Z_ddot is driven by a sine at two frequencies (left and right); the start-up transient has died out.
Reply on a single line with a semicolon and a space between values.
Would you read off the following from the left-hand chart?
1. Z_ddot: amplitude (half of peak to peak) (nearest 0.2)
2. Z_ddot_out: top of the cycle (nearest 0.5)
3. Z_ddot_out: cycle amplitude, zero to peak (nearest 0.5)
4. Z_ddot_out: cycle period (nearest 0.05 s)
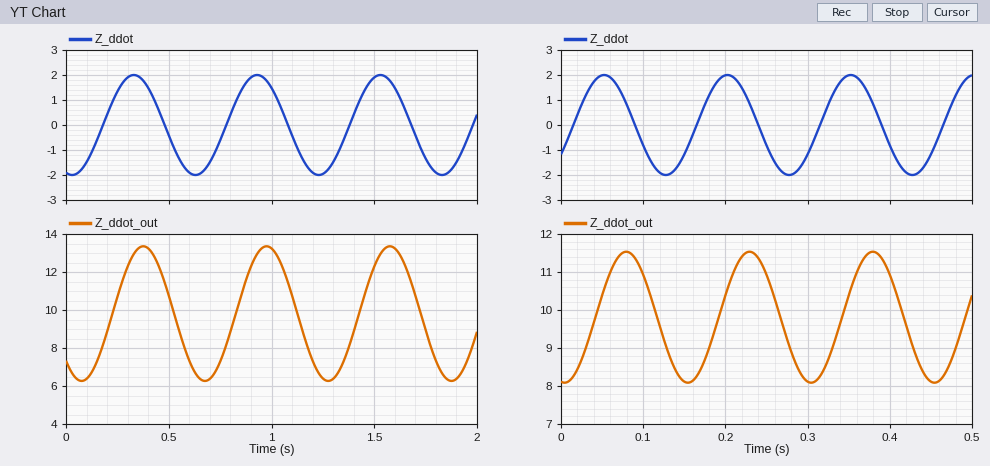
2.0; 13.5; 3.5; 0.60 s
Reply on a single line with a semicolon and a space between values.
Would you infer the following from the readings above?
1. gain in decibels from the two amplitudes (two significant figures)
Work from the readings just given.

4.9 dB
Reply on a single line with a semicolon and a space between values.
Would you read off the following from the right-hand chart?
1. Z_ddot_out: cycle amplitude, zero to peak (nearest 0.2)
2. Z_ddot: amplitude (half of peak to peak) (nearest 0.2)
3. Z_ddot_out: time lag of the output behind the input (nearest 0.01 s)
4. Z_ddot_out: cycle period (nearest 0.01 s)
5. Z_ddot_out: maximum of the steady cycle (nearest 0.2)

1.8; 2.0; 0.03 s; 0.15 s; 11.6
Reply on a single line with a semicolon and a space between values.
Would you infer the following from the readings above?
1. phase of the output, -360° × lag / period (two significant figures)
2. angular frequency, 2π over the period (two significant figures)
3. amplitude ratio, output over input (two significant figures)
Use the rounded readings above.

-72°; 42 rad/s; 0.90
